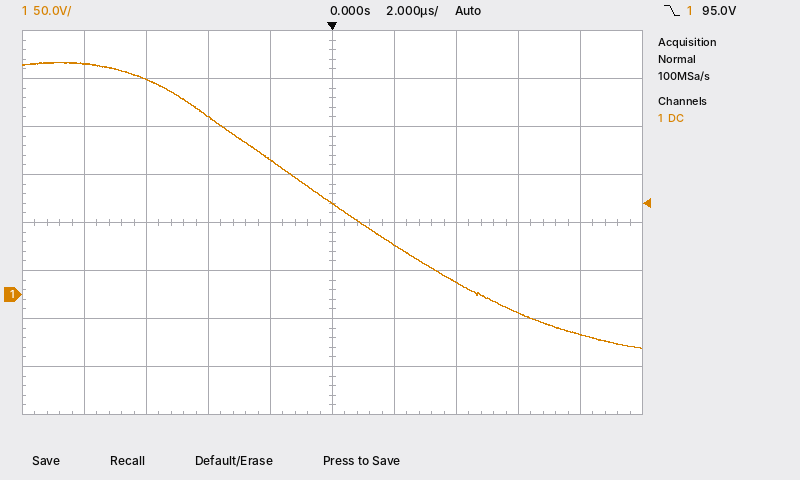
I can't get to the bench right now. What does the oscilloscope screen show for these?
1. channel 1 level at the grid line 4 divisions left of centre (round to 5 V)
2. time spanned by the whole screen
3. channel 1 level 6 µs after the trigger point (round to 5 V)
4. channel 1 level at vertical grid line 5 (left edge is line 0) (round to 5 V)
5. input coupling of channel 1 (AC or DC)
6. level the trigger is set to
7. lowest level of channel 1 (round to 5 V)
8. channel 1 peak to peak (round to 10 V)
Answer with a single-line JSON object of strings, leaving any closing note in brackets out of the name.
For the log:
{"channel 1 level at the grid line 4 divisions left of centre": "240 V", "time spanned by the whole screen": "20 µs", "channel 1 level 6 µs after the trigger point": "-20 V", "channel 1 level at vertical grid line 5 (left edge is line 0)": "95 V", "input coupling of channel 1": "DC", "level the trigger is set to": "95.0 V", "lowest level of channel 1": "-55 V", "channel 1 peak to peak": "300 V"}
